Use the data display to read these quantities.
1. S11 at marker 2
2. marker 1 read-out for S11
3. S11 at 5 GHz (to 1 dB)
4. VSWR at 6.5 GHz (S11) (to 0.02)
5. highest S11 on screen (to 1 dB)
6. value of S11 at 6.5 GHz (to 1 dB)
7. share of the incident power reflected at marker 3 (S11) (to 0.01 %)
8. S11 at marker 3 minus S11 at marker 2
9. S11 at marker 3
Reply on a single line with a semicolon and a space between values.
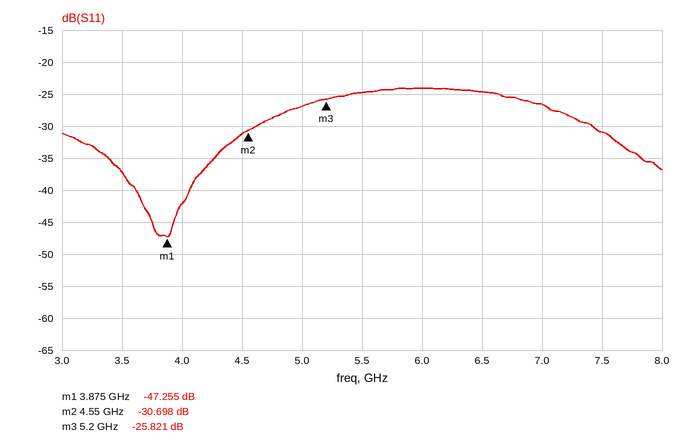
-30.698 dB; -47.255 dB; -27 dB; 1.12; -24 dB; -25 dB; 0.26 %; 4.877 dB; -25.821 dB
